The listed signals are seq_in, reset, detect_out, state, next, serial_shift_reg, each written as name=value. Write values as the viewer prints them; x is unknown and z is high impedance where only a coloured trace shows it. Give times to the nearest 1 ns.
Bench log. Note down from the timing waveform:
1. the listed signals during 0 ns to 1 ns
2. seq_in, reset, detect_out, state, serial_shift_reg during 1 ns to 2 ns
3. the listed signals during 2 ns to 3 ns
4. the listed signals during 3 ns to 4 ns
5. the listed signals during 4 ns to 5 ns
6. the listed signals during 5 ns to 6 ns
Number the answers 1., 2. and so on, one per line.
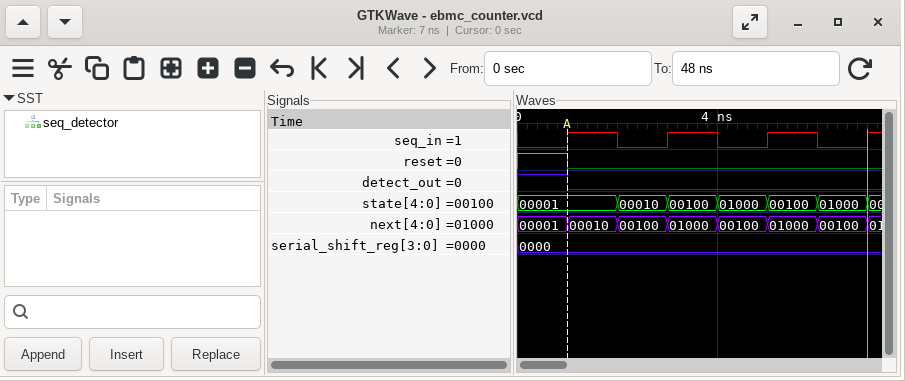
1. seq_in=0, reset=1, detect_out=1, state=00001, next=00001, serial_shift_reg=0000
2. seq_in=1, reset=0, detect_out=0, state=00001, serial_shift_reg=0000
3. seq_in=0, reset=0, detect_out=0, state=00010, next=00100, serial_shift_reg=0000
4. seq_in=1, reset=0, detect_out=0, state=00100, next=01000, serial_shift_reg=0000
5. seq_in=0, reset=0, detect_out=0, state=01000, next=00100, serial_shift_reg=0000
6. seq_in=1, reset=0, detect_out=0, state=00100, next=01000, serial_shift_reg=0000
